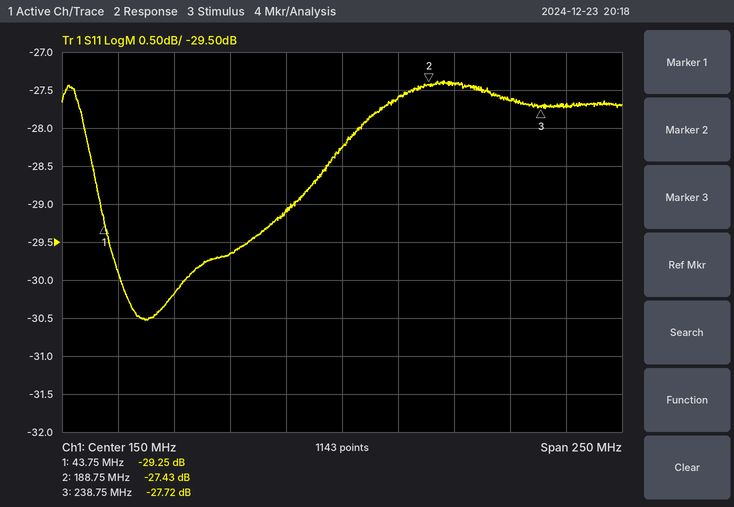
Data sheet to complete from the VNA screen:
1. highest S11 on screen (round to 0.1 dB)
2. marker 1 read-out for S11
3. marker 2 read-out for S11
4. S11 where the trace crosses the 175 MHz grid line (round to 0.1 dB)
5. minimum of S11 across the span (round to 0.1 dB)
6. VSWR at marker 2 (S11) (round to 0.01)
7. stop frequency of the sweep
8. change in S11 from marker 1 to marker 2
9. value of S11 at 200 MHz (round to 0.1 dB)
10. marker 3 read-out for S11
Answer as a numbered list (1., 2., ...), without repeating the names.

1. -27.4 dB
2. -29.25 dB
3. -27.43 dB
4. -27.6 dB
5. -30.5 dB
6. 1.09
7. 275 MHz
8. 1.82 dB
9. -27.4 dB
10. -27.72 dB
